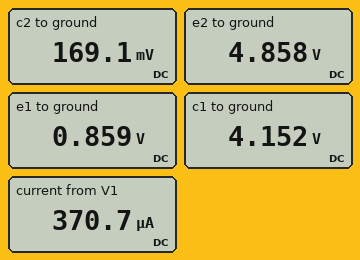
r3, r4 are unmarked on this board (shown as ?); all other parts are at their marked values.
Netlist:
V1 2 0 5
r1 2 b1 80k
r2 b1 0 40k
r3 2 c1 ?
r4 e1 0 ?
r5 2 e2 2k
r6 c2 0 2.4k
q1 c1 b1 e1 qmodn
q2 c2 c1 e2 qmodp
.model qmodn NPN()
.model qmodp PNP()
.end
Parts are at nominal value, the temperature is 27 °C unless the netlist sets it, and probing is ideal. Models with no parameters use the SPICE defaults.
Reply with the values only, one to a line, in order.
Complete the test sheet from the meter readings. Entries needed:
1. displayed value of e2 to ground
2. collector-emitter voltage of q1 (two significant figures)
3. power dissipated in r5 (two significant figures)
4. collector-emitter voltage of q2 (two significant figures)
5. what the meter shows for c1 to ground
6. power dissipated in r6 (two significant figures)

4.858 V
3.3 V
10 µW
-4.7 V
4.152 V
12 µW
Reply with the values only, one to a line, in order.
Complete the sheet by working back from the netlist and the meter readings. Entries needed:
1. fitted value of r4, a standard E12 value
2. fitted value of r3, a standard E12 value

3.3 kΩ
3.3 kΩ
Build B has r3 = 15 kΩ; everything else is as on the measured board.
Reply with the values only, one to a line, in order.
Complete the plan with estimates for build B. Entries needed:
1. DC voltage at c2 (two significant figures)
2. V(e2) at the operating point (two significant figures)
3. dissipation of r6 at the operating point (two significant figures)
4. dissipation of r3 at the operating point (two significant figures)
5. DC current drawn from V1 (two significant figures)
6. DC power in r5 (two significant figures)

2.6 V
2.7 V
2.9 mW
630 µW
1.4 mA
2.6 mW
